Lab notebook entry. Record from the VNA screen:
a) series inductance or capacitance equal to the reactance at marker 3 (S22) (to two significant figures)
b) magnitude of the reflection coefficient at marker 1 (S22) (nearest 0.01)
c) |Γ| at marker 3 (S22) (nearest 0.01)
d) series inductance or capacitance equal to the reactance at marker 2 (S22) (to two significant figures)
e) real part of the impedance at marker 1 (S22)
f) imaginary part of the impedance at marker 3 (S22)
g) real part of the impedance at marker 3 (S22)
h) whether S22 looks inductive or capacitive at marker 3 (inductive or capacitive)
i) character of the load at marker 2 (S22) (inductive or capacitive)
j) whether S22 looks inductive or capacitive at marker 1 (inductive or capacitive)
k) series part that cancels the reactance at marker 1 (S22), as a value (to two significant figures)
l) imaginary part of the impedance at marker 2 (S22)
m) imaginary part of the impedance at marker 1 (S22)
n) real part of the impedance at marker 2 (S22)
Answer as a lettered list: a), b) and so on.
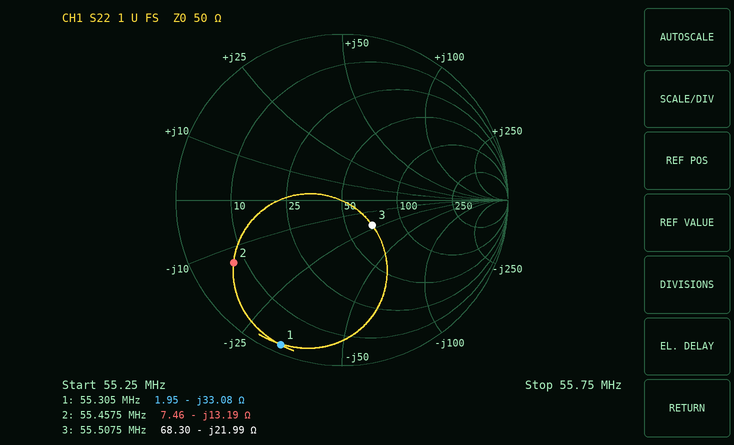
a) 130 pF
b) 0.95
c) 0.24
d) 220 pF
e) 1.95 Ω
f) -21.99 Ω
g) 68.30 Ω
h) capacitive
i) capacitive
j) capacitive
k) 95 nH
l) -13.19 Ω
m) -33.08 Ω
n) 7.46 Ω
